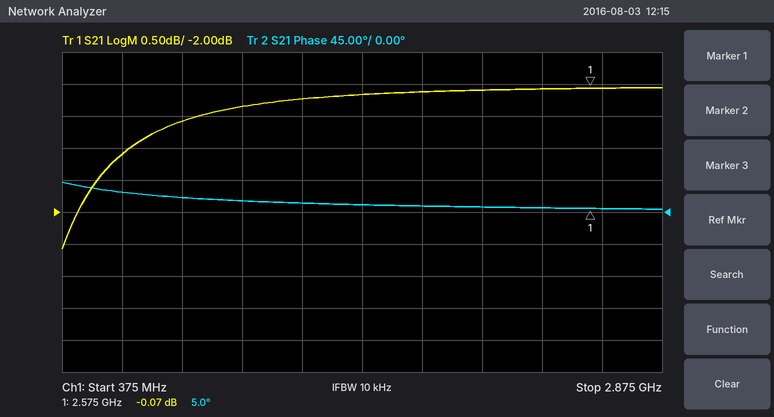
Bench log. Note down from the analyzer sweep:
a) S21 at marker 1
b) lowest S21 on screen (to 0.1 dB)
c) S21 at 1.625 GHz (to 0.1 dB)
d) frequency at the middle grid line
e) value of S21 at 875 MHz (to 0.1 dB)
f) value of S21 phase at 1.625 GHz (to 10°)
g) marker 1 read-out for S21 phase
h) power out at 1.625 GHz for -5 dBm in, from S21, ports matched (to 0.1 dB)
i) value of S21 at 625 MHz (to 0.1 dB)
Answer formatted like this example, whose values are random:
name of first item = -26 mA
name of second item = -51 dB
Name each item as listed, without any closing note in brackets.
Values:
S21 at marker 1 = -0.07 dB
lowest S21 on screen = -2.6 dB
S21 at 1.625 GHz = -0.2 dB
frequency at the middle grid line = 1.625 GHz
value of S21 at 875 MHz = -0.6 dB
value of S21 phase at 1.625 GHz = 10°
marker 1 read-out for S21 phase = 5.0°
power out at 1.625 GHz for -5 dBm in, from S21, ports matched = -5.2 dBm
value of S21 at 625 MHz = -1.1 dB
